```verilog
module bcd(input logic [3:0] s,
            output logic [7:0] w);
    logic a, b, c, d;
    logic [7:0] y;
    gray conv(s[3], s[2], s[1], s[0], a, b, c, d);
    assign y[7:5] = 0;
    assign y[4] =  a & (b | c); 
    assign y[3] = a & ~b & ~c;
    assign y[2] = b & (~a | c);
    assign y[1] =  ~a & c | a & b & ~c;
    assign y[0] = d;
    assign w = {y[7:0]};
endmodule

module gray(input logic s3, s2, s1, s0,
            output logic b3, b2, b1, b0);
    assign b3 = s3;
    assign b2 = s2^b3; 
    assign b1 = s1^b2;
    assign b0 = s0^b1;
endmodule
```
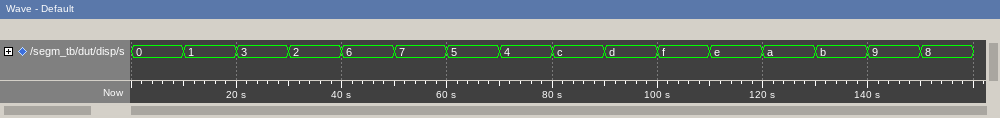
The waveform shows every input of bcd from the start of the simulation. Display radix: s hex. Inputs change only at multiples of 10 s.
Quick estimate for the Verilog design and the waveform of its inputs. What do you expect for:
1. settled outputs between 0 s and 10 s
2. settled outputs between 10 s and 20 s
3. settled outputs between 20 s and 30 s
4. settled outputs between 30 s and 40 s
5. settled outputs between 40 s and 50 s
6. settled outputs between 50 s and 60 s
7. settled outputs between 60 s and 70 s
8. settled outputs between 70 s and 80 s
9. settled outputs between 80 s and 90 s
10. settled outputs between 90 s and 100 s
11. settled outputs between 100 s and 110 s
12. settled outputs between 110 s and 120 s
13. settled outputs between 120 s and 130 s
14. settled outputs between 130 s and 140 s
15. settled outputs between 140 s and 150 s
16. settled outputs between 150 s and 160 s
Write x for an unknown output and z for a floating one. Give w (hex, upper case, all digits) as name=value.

w=00
w=01
w=02
w=03
w=04
w=05
w=06
w=07
w=08
w=09
w=10
w=11
w=12
w=13
w=14
w=15
